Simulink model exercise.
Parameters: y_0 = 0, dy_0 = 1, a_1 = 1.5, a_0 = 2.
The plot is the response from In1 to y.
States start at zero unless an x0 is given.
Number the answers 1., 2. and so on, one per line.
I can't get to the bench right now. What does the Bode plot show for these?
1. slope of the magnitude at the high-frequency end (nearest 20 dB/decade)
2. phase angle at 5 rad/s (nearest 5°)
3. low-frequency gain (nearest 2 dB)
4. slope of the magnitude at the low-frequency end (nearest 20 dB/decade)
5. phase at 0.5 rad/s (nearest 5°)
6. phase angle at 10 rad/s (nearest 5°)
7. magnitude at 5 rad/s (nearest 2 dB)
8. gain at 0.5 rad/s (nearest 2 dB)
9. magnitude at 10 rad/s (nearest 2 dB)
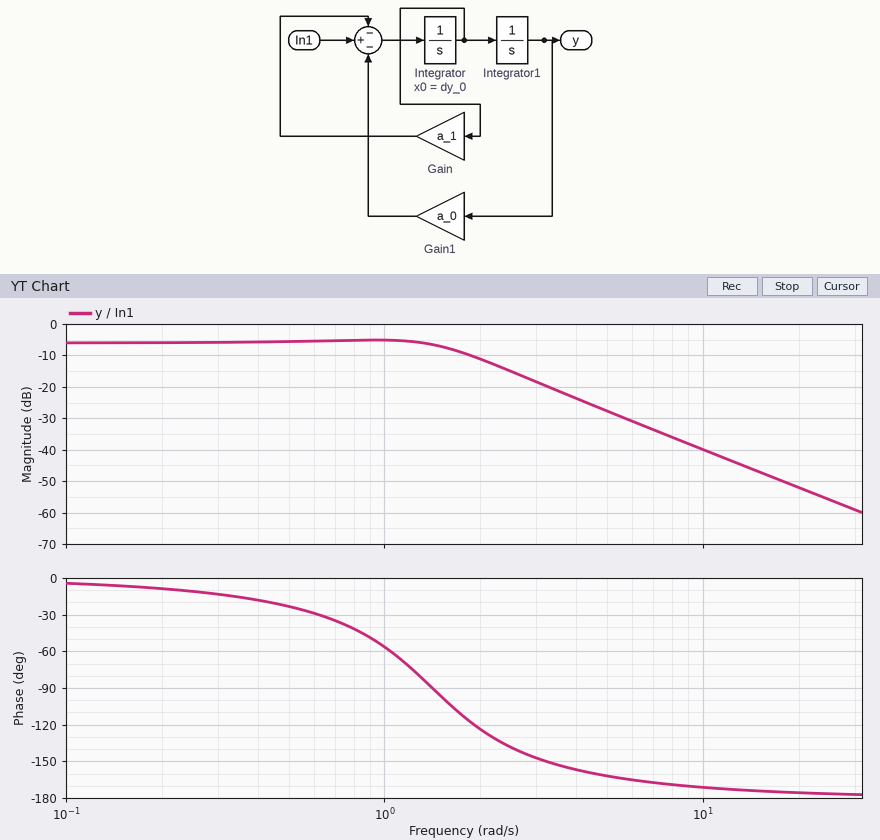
1. -40 dB/decade
2. -160°
3. -6 dB
4. 0 dB/decade
5. -25°
6. -170°
7. -28 dB
8. -6 dB
9. -40 dB
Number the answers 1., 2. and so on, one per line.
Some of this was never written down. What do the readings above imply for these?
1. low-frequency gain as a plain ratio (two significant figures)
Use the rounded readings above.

1. 0.50
